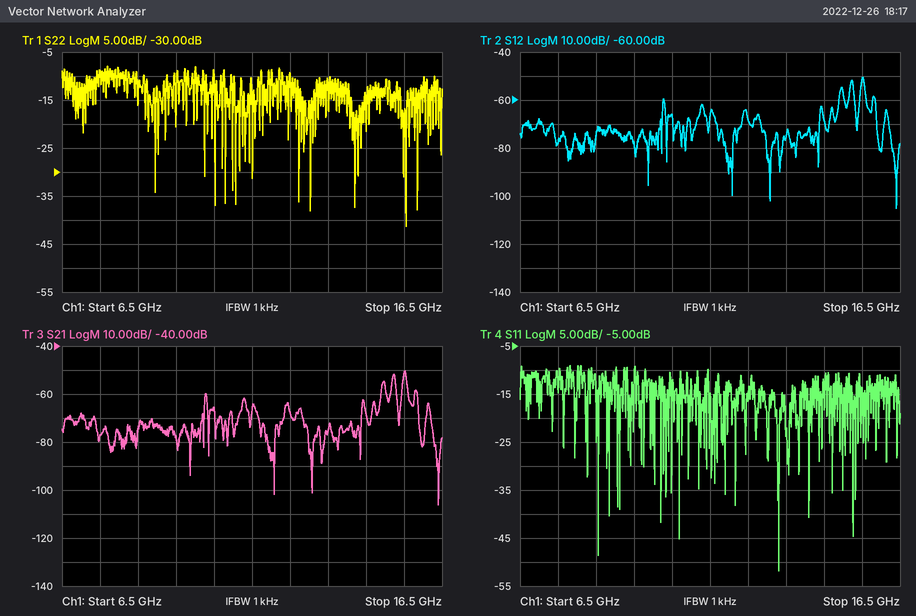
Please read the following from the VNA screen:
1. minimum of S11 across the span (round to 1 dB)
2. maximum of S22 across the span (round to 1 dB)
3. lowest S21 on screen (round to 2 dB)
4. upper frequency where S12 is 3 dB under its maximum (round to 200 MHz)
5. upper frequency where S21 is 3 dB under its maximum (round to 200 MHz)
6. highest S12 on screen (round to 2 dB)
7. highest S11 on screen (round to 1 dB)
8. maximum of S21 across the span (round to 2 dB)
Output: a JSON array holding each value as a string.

["-52 dB", "-8 dB", "-106 dB", "15.6 GHz", "15.6 GHz", "-50 dB", "-9 dB", "-50 dB"]
